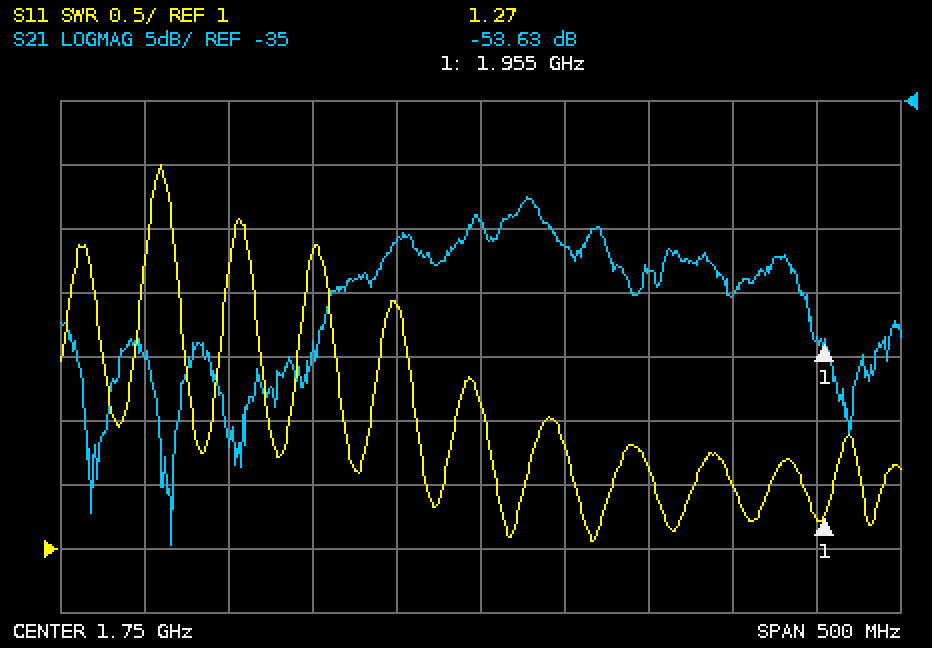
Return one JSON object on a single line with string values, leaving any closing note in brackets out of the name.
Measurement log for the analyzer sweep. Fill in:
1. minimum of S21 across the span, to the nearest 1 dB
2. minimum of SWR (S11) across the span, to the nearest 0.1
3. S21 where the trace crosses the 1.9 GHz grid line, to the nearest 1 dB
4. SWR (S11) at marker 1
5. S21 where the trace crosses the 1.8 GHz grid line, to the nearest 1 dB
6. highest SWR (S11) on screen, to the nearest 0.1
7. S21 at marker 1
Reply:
{"minimum of S21 across the span, to the nearest 1 dB": "-70 dB", "minimum of SWR (S11) across the span, to the nearest 0.1": "1.1", "S21 where the trace crosses the 1.9 GHz grid line, to the nearest 1 dB": "-50 dB", "SWR (S11) at marker 1": "1.27", "S21 where the trace crosses the 1.8 GHz grid line, to the nearest 1 dB": "-46 dB", "highest SWR (S11) on screen, to the nearest 0.1": "4.0", "S21 at marker 1": "-53.63 dB"}
